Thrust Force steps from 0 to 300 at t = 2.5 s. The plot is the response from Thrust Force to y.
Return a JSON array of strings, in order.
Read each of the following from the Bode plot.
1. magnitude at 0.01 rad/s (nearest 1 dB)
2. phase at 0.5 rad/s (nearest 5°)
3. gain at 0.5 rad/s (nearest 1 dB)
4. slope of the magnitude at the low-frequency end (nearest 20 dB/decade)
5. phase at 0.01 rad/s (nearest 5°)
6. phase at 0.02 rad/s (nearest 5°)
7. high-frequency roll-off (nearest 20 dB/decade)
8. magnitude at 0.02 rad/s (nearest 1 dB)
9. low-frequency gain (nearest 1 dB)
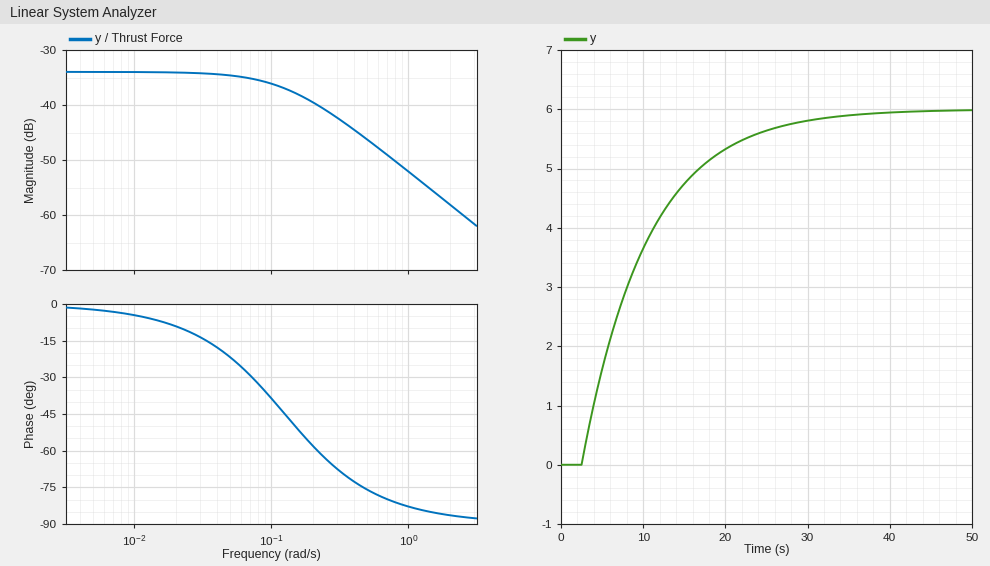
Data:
["-34 dB", "-75°", "-46 dB", "0 dB/decade", "-5°", "-10°", "-20 dB/decade", "-34 dB", "-34 dB"]
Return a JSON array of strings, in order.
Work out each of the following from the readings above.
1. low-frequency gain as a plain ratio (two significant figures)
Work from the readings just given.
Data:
["0.020"]
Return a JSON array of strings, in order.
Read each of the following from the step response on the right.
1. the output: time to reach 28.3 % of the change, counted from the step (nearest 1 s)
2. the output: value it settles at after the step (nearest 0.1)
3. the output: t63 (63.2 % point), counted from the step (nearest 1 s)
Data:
["3 s", "6.0", "8 s"]
